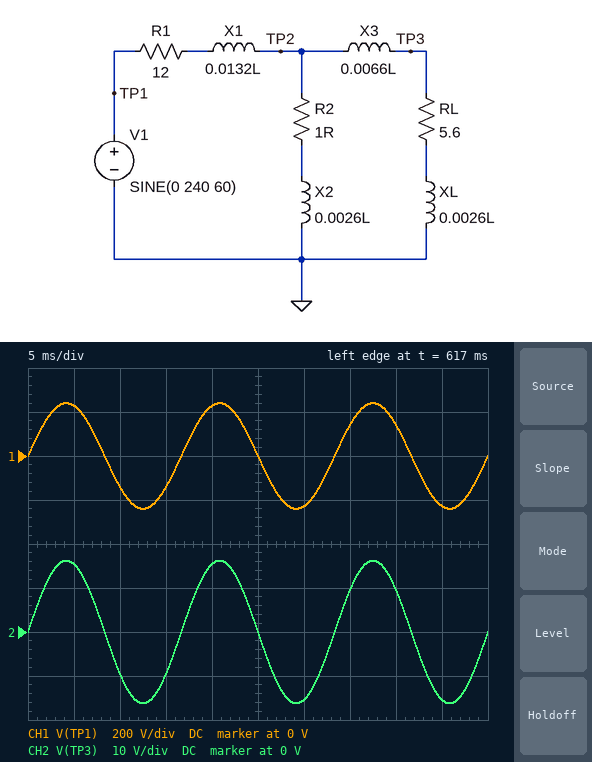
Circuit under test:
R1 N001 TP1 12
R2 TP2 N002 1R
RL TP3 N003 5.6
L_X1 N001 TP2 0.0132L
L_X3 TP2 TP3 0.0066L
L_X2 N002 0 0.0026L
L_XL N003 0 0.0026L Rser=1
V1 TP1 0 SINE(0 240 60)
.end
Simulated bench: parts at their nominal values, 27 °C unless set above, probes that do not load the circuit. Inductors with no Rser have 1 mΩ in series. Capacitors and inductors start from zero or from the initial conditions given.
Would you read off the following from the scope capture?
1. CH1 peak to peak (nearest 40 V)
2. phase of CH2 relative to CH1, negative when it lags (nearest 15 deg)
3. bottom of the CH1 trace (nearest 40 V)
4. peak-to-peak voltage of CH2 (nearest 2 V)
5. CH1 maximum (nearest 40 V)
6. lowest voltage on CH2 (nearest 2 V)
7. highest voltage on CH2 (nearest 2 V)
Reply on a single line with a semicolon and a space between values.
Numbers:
480 V; 0 deg; -240 V; 32 V; 240 V; -16 V; 16 V
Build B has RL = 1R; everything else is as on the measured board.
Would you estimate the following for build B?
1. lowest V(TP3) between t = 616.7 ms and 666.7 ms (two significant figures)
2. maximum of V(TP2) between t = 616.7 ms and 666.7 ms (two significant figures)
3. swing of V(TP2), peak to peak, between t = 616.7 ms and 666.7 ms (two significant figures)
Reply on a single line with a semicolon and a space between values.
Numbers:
-13 V; 13 V; 25 V
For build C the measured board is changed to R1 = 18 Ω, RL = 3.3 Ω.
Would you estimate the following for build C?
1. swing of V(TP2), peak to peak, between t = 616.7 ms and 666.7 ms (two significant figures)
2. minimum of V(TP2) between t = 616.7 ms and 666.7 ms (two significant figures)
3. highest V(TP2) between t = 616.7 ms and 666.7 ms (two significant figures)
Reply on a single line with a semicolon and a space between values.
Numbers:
21 V; -10 V; 10 V
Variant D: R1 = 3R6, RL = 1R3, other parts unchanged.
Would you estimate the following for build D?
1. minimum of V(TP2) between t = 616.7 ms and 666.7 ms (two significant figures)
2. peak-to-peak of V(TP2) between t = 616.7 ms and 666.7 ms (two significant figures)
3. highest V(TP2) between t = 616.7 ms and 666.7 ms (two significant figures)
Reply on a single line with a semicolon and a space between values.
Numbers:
-39 V; 78 V; 39 V
